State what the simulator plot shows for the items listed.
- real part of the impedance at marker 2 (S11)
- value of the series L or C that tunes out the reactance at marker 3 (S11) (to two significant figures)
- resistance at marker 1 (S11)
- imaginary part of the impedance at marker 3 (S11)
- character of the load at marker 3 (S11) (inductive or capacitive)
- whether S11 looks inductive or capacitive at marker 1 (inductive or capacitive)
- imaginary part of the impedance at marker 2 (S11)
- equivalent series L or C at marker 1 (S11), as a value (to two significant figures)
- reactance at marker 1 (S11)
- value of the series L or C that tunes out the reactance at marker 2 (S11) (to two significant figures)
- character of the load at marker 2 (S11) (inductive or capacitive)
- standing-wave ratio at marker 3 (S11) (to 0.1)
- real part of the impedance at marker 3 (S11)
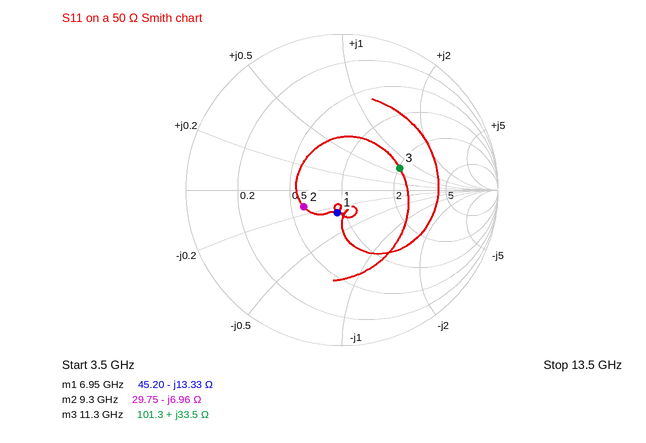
29.75 Ω
420 fF
45.20 Ω
+33.5 Ω
inductive
capacitive
-6.96 Ω
1.7 pF
-13.33 Ω
120 pH
capacitive
2.3
101.3 Ω
